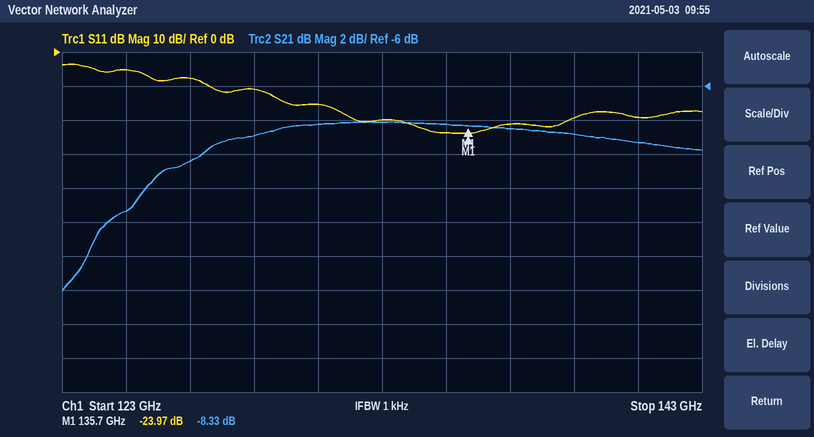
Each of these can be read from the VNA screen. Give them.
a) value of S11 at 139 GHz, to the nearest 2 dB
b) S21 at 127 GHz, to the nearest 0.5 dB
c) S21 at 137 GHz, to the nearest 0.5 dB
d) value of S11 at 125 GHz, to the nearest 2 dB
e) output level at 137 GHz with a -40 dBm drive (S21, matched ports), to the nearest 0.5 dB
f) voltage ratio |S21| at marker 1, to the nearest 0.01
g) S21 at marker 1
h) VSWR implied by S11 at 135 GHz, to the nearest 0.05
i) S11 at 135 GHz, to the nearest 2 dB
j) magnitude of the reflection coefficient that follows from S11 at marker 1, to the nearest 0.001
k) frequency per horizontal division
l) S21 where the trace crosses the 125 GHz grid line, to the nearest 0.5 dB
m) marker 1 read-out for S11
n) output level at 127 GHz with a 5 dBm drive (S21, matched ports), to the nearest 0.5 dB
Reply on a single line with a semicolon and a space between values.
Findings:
-20 dB; -10.5 dB; -8.5 dB; -6 dB; -48.5 dBm; 0.38; -8.33 dB; 1.15; -24 dB; 0.063; 2 GHz; -13.5 dB; -23.97 dB; -5.5 dBm
